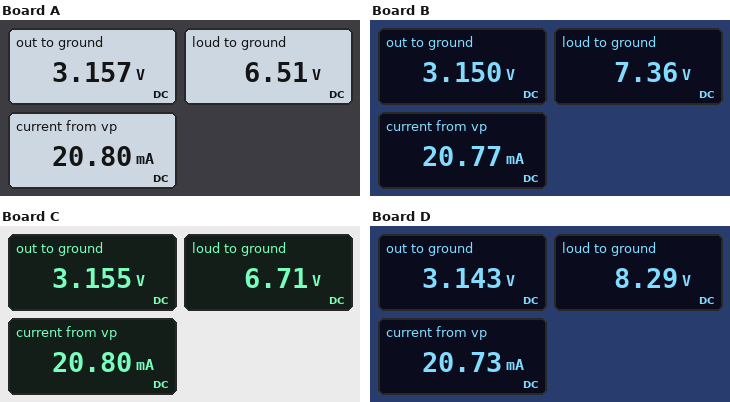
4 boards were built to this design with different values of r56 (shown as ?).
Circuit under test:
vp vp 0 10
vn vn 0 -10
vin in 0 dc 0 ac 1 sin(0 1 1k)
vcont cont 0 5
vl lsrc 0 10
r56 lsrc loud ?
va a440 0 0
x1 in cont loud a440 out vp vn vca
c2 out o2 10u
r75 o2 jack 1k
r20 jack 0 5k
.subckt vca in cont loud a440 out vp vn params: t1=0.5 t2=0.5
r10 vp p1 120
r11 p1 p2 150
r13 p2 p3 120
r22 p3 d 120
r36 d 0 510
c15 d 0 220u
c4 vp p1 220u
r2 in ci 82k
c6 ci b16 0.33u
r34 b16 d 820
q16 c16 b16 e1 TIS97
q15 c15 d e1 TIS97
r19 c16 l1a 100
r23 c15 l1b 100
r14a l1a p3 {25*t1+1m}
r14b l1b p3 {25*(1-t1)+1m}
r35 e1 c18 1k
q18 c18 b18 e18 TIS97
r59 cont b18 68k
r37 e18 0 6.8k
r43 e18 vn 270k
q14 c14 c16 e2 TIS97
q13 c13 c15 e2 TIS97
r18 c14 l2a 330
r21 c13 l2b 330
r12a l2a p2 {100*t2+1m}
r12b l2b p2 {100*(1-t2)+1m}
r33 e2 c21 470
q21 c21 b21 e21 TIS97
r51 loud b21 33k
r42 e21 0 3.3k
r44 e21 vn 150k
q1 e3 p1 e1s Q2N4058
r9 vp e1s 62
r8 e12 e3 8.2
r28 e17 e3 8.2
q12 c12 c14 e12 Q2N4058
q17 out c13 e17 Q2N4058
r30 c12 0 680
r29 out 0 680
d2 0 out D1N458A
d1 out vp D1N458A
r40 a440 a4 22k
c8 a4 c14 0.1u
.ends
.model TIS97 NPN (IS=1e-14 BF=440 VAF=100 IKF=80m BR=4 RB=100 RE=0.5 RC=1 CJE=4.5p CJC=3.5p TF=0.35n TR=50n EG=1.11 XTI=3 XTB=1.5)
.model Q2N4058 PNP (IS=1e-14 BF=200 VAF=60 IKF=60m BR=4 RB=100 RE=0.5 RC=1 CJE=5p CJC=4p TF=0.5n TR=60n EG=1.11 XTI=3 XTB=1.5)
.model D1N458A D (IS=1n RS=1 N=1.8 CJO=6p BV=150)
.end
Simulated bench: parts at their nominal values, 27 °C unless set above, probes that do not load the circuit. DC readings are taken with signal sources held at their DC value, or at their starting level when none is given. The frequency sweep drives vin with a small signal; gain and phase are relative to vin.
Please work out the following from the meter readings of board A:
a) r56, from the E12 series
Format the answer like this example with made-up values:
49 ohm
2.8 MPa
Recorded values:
82 kΩ
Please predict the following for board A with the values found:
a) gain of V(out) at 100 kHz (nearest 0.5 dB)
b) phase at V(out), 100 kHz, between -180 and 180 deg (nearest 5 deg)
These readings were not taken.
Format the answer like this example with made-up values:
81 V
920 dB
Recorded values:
6.0 dB
-5 deg
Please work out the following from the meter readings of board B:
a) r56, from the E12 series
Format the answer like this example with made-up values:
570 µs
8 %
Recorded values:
39 kΩ
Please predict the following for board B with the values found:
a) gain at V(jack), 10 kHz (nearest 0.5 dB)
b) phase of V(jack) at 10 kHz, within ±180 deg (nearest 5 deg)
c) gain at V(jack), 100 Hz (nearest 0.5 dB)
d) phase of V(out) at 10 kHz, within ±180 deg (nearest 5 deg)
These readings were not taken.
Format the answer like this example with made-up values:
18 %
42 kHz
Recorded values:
4.0 dB
0 deg
4.0 dB
0 deg
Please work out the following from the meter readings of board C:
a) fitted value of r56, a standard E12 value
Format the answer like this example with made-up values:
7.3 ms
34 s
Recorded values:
68 kΩ
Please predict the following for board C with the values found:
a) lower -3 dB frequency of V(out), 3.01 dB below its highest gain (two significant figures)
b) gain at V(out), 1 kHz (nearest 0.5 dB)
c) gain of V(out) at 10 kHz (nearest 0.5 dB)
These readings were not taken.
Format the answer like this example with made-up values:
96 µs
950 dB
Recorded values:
5.6 Hz
6.0 dB
6.0 dB
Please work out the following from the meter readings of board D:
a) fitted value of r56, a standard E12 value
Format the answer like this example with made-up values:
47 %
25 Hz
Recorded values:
18 kΩ
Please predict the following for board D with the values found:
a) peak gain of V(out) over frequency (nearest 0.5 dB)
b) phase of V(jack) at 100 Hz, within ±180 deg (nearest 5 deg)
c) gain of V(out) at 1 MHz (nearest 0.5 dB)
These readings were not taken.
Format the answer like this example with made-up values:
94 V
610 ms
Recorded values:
5.5 dB
5 deg
5.0 dB
